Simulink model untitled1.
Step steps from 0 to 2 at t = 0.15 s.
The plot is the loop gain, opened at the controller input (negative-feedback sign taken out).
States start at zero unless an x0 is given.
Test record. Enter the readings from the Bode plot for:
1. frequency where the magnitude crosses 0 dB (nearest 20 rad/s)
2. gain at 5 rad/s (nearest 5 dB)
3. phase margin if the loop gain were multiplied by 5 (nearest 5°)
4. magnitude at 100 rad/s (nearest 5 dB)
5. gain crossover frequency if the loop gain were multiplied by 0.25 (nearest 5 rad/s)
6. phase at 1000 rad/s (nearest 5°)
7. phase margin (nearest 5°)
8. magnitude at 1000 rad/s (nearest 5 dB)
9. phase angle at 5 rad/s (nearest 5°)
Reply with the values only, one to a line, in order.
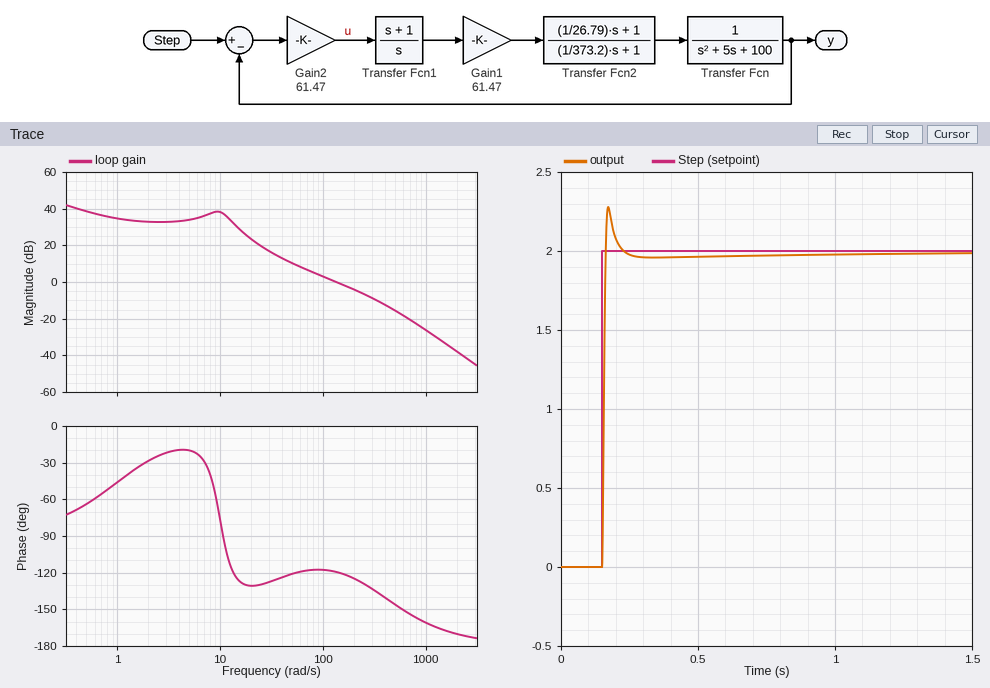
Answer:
140 rad/s
35 dB
35°
5 dB
45 rad/s
-160°
60°
-25 dB
-20°
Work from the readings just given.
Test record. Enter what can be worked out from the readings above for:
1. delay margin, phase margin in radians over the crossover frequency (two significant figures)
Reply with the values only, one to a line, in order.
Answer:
0.0075 s
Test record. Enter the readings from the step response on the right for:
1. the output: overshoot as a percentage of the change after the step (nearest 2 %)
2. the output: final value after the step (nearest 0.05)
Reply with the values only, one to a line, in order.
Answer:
14 %
2.00
